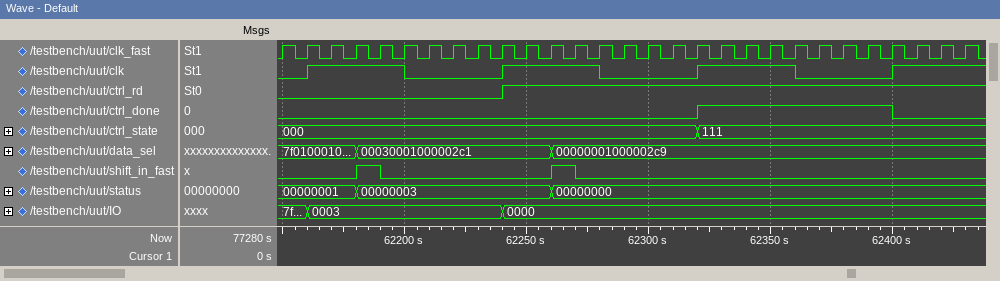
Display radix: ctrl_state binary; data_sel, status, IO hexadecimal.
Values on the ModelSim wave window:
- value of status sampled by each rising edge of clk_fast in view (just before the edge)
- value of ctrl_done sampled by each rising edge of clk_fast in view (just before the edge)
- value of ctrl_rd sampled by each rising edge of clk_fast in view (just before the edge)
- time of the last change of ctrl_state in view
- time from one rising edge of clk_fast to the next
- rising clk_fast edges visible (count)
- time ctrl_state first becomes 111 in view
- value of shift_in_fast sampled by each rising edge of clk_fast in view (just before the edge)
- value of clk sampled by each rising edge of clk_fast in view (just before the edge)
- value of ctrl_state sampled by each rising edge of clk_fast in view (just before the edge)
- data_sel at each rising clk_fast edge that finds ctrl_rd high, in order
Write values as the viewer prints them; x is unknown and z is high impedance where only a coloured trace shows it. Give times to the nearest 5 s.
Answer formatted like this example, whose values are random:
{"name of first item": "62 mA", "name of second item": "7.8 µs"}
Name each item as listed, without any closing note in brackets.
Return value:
{"value of status sampled by each rising edge of clk_fast in view": "00000001, 00000001, 00000001, 00000001, 00000003, 00000003, 00000003, 00000003, 00000003, 00000003, 00000003, 00000003, 00000000, 00000000, 00000000, 00000000, 00000000, 00000000, 00000000, 00000000, 00000000, 00000000, 00000000, 00000000, 00000000, 00000000, 00000000, 00000000, 00000000", "value of ctrl_done sampled by each rising edge of clk_fast in view": "0 0 0 0 0 0 0 0 0 0 0 0 0 0 0 0 0 0 1 1 1 1 1 1 1 1 0 0 0", "value of ctrl_rd sampled by each rising edge of clk_fast in view": "0 0 0 0 0 0 0 0 0 0 1 1 1 1 1 1 1 1 1 1 1 1 1 1 1 1 1 1 1", "time of the last change of ctrl_state in view": "62320 s", "time from one rising edge of clk_fast to the next": "10 s", "rising clk_fast edges visible": "29", "time ctrl_state first becomes 111 in view": "62320 s", "value of shift_in_fast sampled by each rising edge of clk_fast in view": "0 0 0 0 1 0 0 0 0 0 0 0 1 0 0 0 0 0 0 0 0 0 0 0 0 0 0 0 0", "value of clk sampled by each rising edge of clk_fast in view": "0 0 1 1 1 1 0 0 0 0 1 1 1 1 0 0 0 0 1 1 1 1 0 0 0 0 1 1 1", "value of ctrl_state sampled by each rising edge of clk_fast in view": "000, 000, 000, 000, 000, 000, 000, 000, 000, 000, 000, 000, 000, 000, 000, 000, 000, 000, 111, 111, 111, 111, 111, 111, 111, 111, 111, 111, 111", "data_sel at each rising clk_fast edge that finds ctrl_rd high, in order": "00030001000002c1, 00030001000002c1, 00000001000002c9, 00000001000002c9, 00000001000002c9, 00000001000002c9, 00000001000002c9, 00000001000002c9, 00000001000002c9, 00000001000002c9, 00000001000002c9, 00000001000002c9, 00000001000002c9, 00000001000002c9, 00000001000002c9, 00000001000002c9, 00000001000002c9, 00000001000002c9, 00000001000002c9"}
